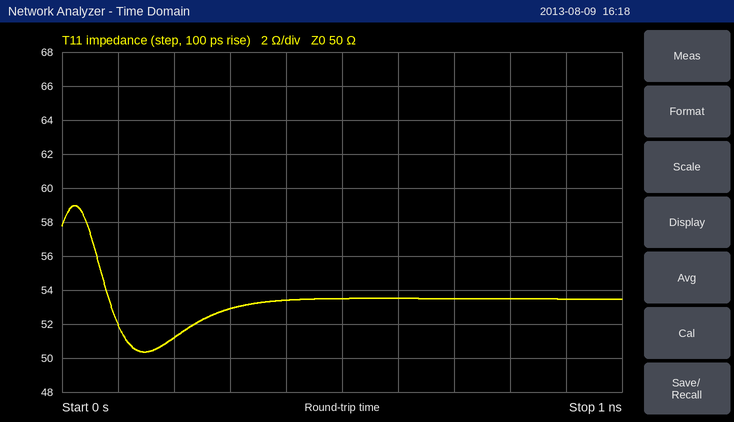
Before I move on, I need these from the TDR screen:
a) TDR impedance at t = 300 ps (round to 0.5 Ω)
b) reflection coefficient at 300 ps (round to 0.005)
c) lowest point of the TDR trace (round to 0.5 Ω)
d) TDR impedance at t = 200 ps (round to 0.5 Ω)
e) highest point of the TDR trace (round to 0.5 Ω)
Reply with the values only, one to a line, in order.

53.0 Ω
+0.030
50.5 Ω
51.0 Ω
59.0 Ω
